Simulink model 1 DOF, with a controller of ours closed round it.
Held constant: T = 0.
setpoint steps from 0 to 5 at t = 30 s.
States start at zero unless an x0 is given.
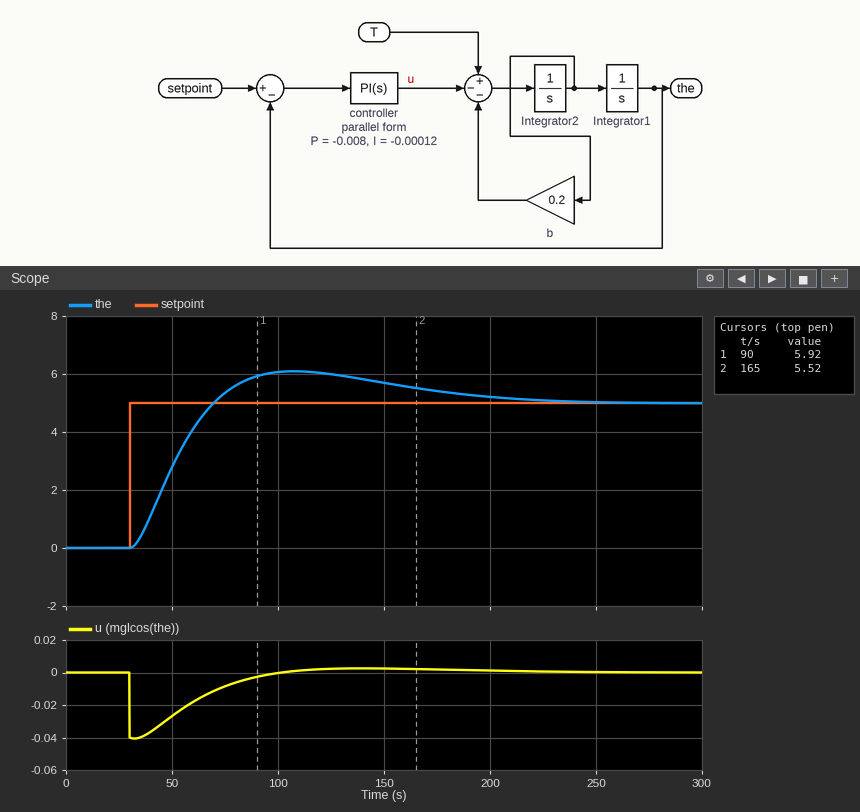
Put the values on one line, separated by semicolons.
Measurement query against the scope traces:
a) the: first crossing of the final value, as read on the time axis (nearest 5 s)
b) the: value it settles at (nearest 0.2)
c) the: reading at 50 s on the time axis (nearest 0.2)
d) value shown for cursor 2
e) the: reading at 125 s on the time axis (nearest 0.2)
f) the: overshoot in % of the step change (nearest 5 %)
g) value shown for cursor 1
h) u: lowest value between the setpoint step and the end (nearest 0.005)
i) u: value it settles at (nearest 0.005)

70 s; 5.0; 2.8; 5.52; 6.0; 20 %; 5.92; -0.040; 0.000
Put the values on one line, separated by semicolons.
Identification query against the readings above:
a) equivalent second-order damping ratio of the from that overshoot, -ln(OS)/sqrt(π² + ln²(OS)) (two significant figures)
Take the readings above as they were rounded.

0.46
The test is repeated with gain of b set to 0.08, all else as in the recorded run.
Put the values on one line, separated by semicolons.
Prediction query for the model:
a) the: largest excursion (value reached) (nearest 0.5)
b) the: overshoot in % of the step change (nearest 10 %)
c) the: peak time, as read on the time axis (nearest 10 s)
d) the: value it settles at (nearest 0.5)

7.0; 40 %; 70 s; 5.0
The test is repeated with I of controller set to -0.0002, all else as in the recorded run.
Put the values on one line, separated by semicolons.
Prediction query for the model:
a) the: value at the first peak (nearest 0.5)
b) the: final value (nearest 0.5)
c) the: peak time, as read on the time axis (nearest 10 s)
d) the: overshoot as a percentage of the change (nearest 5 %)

6.5; 5.0; 100 s; 30 %
